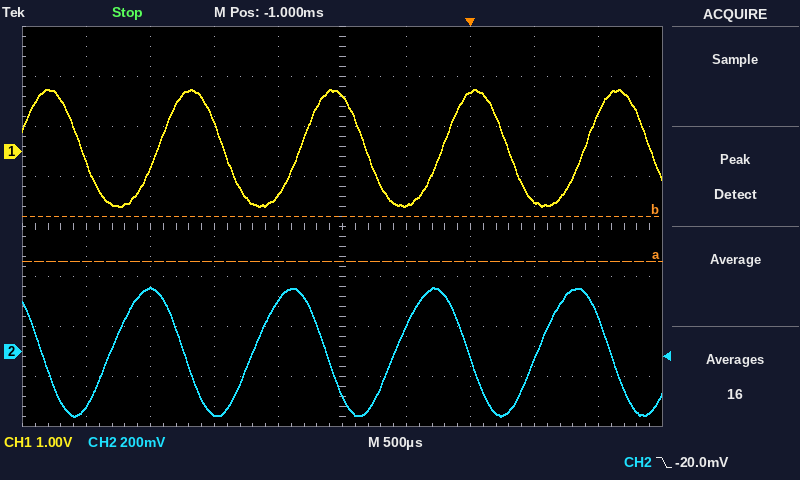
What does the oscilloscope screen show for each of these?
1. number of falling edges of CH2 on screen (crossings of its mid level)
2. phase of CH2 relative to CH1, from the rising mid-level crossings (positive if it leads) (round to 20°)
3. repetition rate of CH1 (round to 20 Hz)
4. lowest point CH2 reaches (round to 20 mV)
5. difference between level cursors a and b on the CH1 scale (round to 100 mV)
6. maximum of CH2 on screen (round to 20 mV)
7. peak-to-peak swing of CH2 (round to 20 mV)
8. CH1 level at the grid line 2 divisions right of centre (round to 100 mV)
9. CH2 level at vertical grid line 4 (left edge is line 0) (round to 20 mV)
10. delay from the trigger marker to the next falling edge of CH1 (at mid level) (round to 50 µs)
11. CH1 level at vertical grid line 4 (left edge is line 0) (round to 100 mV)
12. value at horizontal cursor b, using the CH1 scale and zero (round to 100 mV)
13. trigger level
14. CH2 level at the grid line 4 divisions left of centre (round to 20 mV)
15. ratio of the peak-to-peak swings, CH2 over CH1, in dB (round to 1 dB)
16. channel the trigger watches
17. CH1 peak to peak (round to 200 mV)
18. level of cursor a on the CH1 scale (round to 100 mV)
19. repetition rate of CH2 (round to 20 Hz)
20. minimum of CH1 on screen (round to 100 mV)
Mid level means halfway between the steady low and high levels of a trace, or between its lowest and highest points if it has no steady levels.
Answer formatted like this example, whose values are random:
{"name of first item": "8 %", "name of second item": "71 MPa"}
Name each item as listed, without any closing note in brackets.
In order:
{"number of falling edges of CH2 on screen": "5", "phase of CH2 relative to CH1, from the rising mid-level crossings (positive if it leads)": "+120°", "repetition rate of CH1": "900 Hz", "lowest point CH2 reaches": "-260 mV", "difference between level cursors a and b on the CH1 scale": "900 mV", "maximum of CH2 on screen": "260 mV", "peak-to-peak swing of CH2": "520 mV", "CH1 level at the grid line 2 divisions right of centre": "1.2 V", "CH2 level at vertical grid line 4 (left edge is line 0)": "200 mV", "delay from the trigger marker to the next falling edge of CH1 (at mid level)": "300 µs", "CH1 level at vertical grid line 4 (left edge is line 0)": "-900 mV", "value at horizontal cursor b, using the CH1 scale and zero": "-1.3 V", "trigger level": "-20.0 mV", "CH2 level at the grid line 4 divisions left of centre": "-220 mV", "ratio of the peak-to-peak swings, CH2 over CH1, in dB": "-13 dB", "channel the trigger watches": "CH2", "CH1 peak to peak": "2.4 V", "level of cursor a on the CH1 scale": "-2.2 V", "repetition rate of CH2": "900 Hz", "minimum of CH1 on screen": "-1.1 V"}
